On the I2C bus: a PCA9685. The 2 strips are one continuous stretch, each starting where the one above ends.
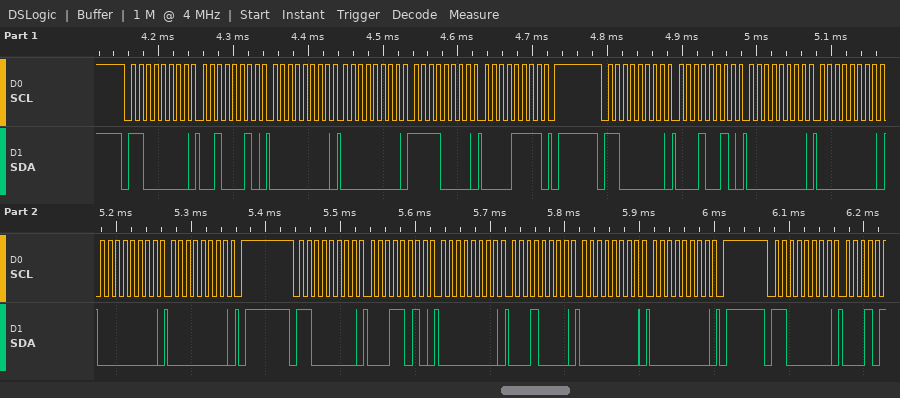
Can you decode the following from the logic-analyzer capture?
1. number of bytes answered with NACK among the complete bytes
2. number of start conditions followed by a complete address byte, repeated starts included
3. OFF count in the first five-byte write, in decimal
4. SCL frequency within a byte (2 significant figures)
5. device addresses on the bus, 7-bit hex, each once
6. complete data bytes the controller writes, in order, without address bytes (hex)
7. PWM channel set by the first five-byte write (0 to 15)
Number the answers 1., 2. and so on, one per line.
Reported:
1. 0
2. 4
3. 4080
4. 100 kHz
5. 0x60
6. 22 00 00 F0 0F 12 00 00 00 00 1A 00 10 00 00
7. 7
